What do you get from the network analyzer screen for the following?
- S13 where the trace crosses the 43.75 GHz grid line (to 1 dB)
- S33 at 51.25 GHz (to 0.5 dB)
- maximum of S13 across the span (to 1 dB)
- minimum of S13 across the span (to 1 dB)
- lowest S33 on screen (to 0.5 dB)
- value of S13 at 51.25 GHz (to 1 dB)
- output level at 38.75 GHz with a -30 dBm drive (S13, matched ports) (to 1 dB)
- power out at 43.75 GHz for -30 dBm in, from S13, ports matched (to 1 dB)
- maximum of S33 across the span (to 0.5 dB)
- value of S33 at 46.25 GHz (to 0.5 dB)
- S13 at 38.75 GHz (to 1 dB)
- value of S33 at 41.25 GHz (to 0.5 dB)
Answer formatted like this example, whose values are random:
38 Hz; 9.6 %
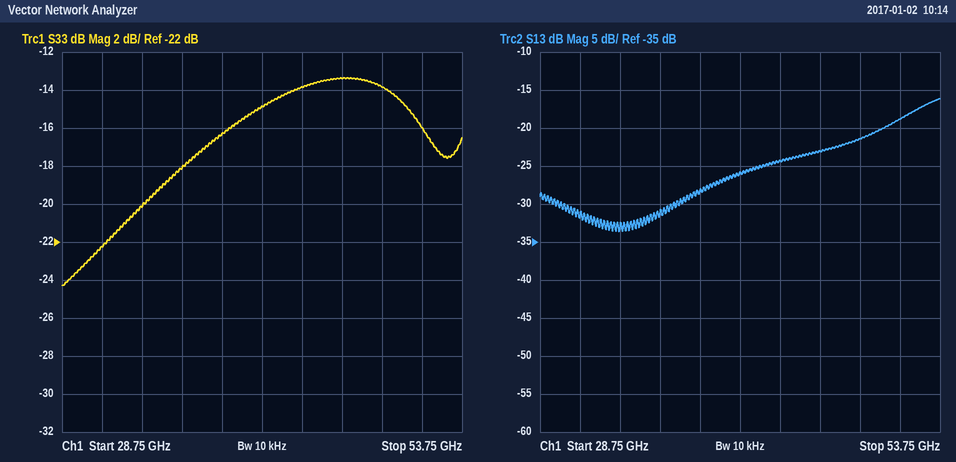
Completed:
-24 dB; -16.0 dB; -16 dB; -34 dB; -24.5 dB; -19 dB; -58 dBm; -54 dBm; -13.5 dB; -13.5 dB; -28 dB; -15.0 dB
